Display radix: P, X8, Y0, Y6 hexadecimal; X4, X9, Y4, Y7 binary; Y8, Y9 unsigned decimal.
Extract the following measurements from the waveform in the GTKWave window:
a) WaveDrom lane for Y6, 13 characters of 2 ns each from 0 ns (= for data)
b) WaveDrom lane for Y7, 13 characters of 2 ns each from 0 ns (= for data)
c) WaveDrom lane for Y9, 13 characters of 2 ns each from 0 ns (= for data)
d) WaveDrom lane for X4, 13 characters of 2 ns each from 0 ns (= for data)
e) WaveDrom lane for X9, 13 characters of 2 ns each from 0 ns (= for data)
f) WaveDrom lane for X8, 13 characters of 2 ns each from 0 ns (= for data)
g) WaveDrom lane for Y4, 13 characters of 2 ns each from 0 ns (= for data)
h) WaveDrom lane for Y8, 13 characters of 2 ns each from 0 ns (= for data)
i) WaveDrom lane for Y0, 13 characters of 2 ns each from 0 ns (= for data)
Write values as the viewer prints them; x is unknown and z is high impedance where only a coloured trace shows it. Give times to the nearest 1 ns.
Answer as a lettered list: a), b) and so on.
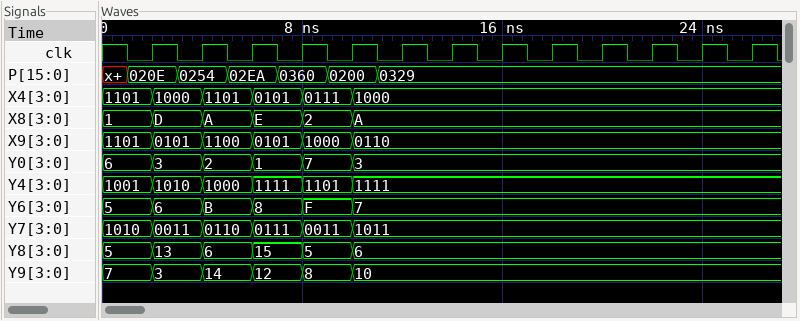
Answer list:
a) {name: 'Y6', wave: '======.......', data: '5 6 B 8 F 7'}
b) {name: 'Y7', wave: '======.......', data: '1010 0011 0110 0111 0011 1011'}
c) {name: 'Y9', wave: '======.......', data: '7 3 14 12 8 10'}
d) {name: 'X4', wave: '======.......', data: '1101 1000 1101 0101 0111 1000'}
e) {name: 'X9', wave: '======.......', data: '1101 0101 1100 0101 1000 0110'}
f) {name: 'X8', wave: '======.......', data: '1 D A E 2 A'}
g) {name: 'Y4', wave: '======.......', data: '1001 1010 1000 1111 1101 1111'}
h) {name: 'Y8', wave: '======.......', data: '5 13 6 15 5 6'}
i) {name: 'Y0', wave: '======.......', data: '6 3 2 1 7 3'}
